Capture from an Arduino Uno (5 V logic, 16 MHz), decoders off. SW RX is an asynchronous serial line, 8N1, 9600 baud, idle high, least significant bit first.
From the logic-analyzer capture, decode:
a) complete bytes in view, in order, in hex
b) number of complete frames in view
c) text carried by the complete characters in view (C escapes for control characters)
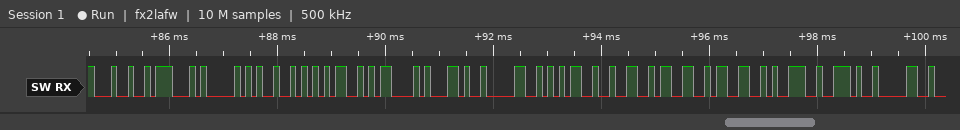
0x24 0x47 0x50 0x52 0x4D 0x43 0x2C 0x30 0x35 0x32 0x33 0x33 0x39 0x2E 0x30
15
"$GPRMC,052339.0"
